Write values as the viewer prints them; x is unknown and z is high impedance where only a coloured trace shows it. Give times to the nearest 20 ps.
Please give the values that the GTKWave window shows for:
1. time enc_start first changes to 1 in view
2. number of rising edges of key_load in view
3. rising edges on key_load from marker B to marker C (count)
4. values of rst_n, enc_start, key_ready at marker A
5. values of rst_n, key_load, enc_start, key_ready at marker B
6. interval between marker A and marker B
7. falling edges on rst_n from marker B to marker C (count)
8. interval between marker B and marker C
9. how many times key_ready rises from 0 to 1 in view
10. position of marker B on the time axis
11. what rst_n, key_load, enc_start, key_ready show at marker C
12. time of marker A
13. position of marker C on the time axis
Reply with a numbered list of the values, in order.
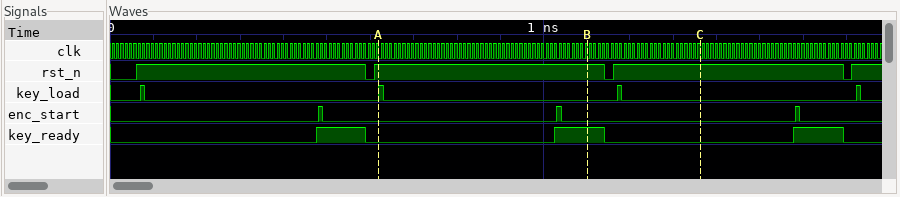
1. 480 ps
2. 4
3. 1
4. rst_n=1, enc_start=0, key_ready=0
5. rst_n=1, key_load=0, enc_start=0, key_ready=1
6. 480 ps
7. 1
8. 260 ps
9. 3
10. 1100 ps
11. rst_n=1, key_load=0, enc_start=0, key_ready=0
12. 620 ps
13. 1360 ps
